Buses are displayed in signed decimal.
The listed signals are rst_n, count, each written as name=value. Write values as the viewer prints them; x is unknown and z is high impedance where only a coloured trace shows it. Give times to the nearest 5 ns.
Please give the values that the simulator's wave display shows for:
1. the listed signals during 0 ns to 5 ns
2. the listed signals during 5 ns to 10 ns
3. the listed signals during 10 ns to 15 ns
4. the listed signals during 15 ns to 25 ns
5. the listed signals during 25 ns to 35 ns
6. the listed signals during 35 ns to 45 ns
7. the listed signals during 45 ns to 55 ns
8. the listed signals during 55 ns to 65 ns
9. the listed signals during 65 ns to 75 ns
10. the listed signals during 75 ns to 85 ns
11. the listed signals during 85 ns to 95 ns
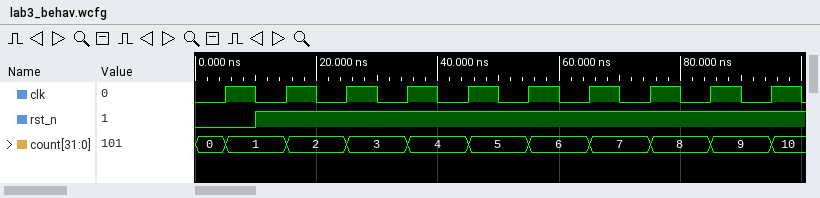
rst_n=0, count=0
rst_n=0, count=1
rst_n=1, count=1
rst_n=1, count=2
rst_n=1, count=3
rst_n=1, count=4
rst_n=1, count=5
rst_n=1, count=6
rst_n=1, count=7
rst_n=1, count=8
rst_n=1, count=9
